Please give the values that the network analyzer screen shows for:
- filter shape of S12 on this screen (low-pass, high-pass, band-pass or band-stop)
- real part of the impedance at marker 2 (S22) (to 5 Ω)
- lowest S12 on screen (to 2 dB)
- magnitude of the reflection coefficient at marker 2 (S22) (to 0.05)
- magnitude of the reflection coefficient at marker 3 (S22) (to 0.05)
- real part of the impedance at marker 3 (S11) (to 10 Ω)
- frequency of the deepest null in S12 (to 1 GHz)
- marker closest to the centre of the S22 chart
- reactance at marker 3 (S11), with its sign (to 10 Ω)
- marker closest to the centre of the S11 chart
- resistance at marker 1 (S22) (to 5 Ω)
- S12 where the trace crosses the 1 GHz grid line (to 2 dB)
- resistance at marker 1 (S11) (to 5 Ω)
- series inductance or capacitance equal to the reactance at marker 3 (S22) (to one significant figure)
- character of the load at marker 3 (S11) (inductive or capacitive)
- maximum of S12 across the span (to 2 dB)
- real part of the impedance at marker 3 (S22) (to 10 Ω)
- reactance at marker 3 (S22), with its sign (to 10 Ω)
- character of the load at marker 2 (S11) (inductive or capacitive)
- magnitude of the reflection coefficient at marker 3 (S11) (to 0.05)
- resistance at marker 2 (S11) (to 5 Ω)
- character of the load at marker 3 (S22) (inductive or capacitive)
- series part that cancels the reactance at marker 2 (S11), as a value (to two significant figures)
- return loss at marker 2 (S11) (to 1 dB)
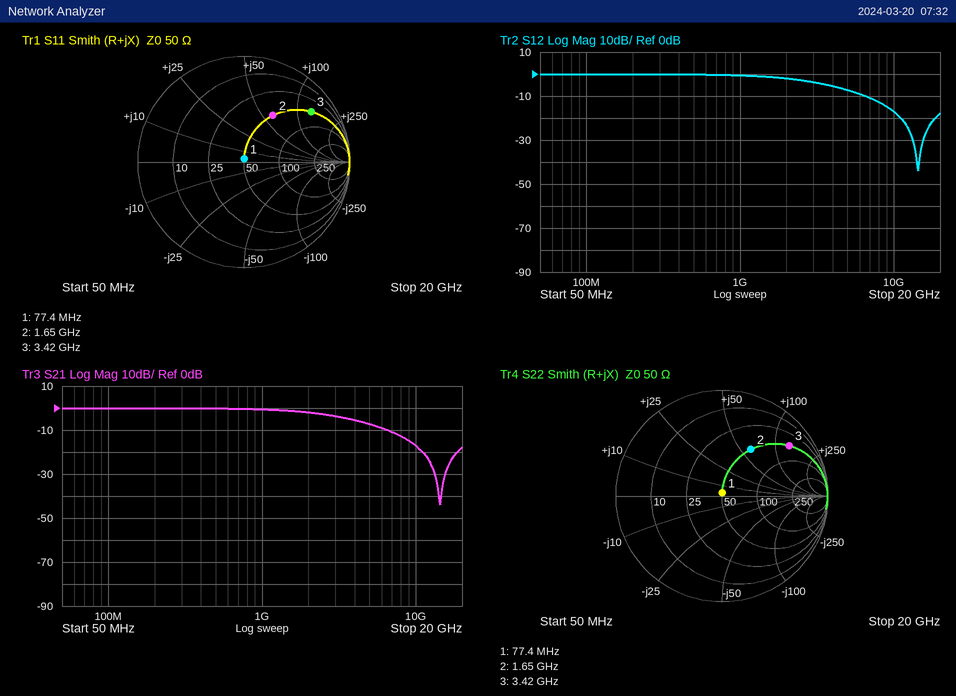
low-pass
50 Ω
-44 dB
0.50
0.80
50 Ω
14 GHz
marker 1
+130 Ω
marker 1
50 Ω
0 dB
50 Ω
6 nH
inductive
0 dB
50 Ω
+130 Ω
inductive
0.80
50 Ω
inductive
1.6 pF
6 dB
